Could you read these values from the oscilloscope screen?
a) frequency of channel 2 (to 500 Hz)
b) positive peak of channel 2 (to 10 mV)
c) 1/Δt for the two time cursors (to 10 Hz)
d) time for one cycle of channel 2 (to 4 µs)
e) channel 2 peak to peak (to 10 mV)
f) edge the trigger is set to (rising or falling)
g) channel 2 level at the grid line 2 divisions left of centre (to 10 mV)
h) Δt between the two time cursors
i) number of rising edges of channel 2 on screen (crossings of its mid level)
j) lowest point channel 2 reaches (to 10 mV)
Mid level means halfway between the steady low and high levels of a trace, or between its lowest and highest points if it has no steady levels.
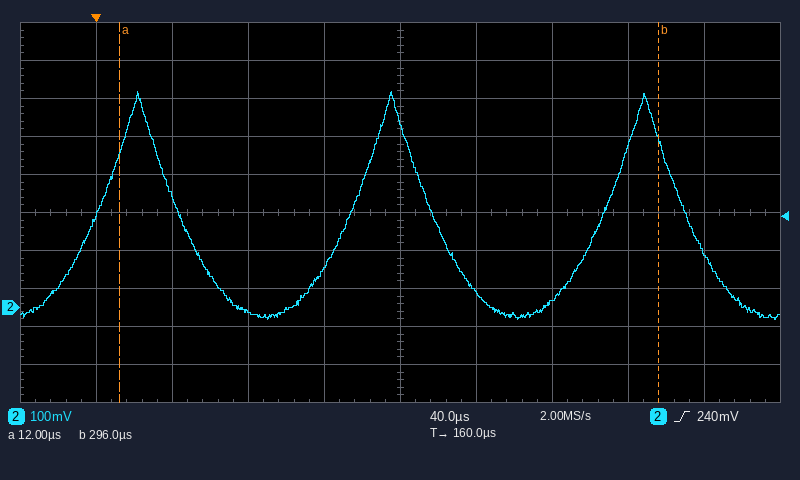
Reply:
7.5 kHz
570 mV
3.52 kHz
132 µs
600 mV
rising
-10 mV
284 µs
3
-30 mV
